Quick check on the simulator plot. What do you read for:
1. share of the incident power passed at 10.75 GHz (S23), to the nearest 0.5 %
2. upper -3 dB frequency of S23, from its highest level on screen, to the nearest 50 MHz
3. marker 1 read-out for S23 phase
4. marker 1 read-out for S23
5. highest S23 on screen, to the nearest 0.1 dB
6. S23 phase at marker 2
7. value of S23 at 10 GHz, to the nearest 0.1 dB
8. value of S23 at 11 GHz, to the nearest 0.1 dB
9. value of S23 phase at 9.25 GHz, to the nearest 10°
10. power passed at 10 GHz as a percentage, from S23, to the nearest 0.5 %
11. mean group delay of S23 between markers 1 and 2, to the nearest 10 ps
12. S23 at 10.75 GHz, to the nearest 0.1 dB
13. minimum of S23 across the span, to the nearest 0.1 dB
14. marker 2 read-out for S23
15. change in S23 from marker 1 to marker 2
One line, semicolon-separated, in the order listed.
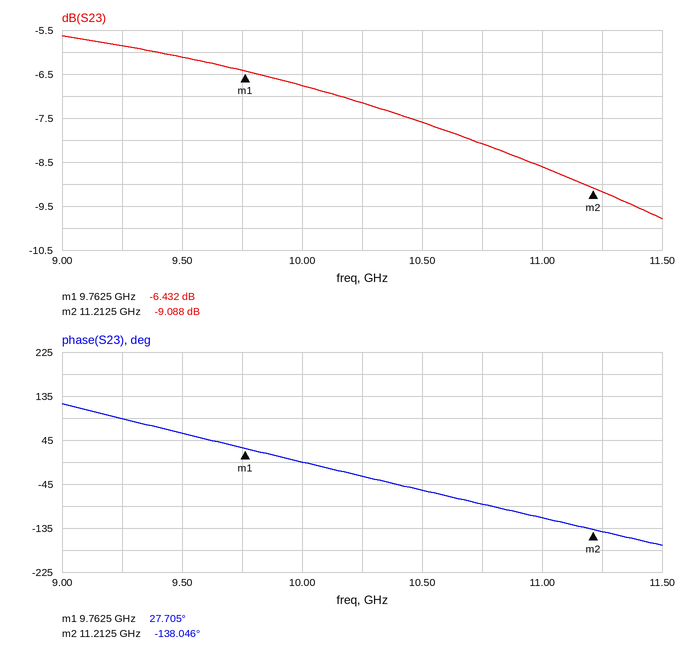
15.5 %; 11.00 GHz; 27.705°; -6.432 dB; -5.6 dB; -138.046°; -6.8 dB; -8.6 dB; 90°; 21.0 %; 320 ps; -8.1 dB; -9.8 dB; -9.088 dB; -2.656 dB
